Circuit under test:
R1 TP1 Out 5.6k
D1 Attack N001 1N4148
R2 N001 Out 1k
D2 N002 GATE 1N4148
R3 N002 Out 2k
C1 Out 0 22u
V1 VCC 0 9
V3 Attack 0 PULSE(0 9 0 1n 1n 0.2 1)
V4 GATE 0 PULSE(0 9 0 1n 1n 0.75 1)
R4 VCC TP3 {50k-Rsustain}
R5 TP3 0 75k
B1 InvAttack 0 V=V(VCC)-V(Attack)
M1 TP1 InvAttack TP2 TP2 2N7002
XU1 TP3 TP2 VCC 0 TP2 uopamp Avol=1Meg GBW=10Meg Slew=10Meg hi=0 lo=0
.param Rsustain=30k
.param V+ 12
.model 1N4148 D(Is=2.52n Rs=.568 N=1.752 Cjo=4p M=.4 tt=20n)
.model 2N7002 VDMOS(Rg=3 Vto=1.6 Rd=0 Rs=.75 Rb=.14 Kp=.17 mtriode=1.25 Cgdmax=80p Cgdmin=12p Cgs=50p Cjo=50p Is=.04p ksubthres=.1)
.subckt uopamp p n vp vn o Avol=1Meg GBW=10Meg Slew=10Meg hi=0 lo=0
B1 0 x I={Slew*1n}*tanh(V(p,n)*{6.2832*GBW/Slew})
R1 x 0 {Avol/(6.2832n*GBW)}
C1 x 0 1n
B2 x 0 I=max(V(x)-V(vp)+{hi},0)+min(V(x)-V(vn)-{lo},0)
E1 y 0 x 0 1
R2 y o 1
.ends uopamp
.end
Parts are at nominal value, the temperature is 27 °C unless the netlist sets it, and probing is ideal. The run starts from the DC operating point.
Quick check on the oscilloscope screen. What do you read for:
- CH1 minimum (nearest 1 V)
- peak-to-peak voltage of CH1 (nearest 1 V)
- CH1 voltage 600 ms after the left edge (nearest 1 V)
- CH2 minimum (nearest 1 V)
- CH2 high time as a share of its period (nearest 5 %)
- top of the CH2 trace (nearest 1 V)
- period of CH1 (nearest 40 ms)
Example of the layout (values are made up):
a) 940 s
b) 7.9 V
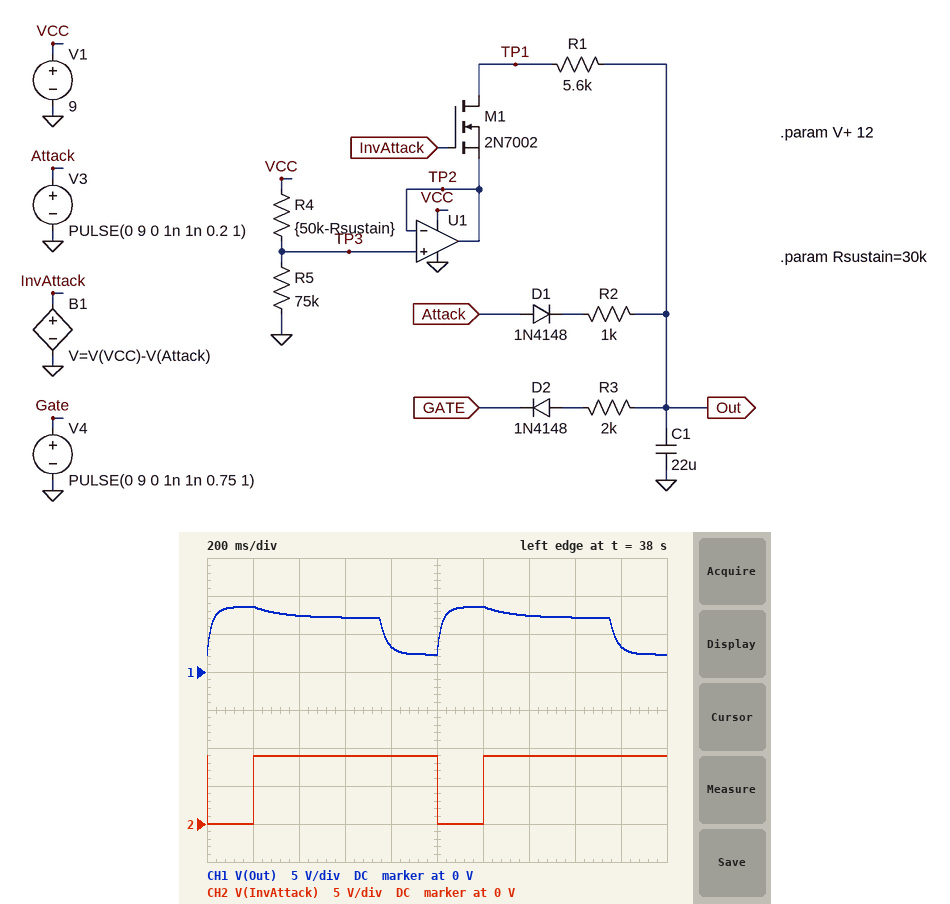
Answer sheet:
a) 2 V
b) 6 V
c) 7 V
d) 0 V
e) 80 %
f) 9 V
g) 1.00 s
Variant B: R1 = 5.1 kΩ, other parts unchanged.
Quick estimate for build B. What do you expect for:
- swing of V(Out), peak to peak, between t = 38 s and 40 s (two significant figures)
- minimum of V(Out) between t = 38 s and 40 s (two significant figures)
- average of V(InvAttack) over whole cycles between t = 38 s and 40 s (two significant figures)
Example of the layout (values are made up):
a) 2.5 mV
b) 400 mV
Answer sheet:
a) 6.2 V
b) 2.4 V
c) 7.2 V
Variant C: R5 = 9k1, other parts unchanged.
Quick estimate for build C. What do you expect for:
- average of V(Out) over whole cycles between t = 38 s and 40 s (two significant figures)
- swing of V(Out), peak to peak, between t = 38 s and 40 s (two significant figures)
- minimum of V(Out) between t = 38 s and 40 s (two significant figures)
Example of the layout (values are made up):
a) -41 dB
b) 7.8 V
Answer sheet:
a) 4.1 V
b) 7.5 V
c) 1.1 V
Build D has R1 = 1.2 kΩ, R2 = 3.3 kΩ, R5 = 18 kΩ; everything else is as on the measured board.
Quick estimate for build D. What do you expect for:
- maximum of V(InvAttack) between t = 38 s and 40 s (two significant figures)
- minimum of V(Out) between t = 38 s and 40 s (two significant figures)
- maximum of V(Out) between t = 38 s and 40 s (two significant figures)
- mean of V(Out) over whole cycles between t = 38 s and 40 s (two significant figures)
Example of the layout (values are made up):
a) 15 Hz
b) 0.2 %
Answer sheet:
a) 9.0 V
b) 2.9 V
c) 8.1 V
d) 4.5 V
